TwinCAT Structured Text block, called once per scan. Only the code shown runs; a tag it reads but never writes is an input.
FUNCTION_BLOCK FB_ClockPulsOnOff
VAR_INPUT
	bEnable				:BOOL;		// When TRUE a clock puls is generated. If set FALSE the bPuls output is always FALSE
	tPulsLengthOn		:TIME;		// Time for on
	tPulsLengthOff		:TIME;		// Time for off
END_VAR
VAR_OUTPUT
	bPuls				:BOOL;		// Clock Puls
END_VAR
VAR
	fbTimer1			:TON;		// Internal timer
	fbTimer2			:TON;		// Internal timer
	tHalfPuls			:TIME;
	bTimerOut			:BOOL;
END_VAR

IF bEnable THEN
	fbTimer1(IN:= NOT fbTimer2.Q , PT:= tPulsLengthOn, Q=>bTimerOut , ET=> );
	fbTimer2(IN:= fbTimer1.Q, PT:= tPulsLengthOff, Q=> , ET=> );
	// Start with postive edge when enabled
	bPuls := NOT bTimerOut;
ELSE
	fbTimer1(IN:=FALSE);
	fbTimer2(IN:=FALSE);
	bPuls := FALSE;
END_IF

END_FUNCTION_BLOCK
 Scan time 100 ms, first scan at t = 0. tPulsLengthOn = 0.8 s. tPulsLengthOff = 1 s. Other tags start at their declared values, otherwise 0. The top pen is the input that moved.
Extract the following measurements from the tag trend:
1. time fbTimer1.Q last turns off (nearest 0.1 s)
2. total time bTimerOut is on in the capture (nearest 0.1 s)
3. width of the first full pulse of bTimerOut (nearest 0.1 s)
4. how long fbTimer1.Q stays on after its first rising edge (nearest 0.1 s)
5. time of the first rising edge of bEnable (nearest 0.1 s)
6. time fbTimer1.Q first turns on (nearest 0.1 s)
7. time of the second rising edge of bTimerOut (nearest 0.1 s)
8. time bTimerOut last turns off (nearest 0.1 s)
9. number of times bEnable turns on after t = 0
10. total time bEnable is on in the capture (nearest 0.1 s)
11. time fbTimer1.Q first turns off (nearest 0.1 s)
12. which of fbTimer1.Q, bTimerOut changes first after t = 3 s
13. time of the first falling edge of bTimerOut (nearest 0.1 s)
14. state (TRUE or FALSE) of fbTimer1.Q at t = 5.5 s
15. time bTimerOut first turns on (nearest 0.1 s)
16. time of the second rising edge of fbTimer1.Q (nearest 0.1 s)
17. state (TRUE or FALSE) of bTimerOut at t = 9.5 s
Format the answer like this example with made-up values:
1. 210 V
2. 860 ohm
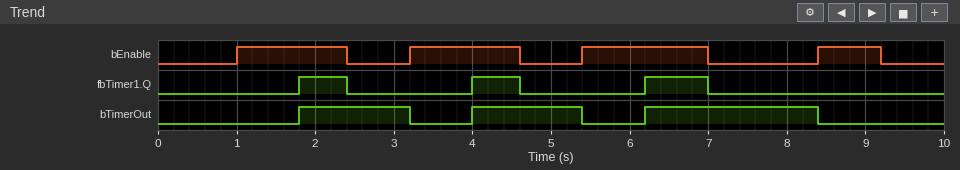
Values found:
1. 7.0 s
2. 5.0 s
3. 1.4 s
4. 0.6 s
5. 1.0 s
6. 1.8 s
7. 4.0 s
8. 8.4 s
9. 4
10. 5.2 s
11. 2.4 s
12. bTimerOut
13. 3.2 s
14. FALSE
15. 1.8 s
16. 4.0 s
17. FALSE
